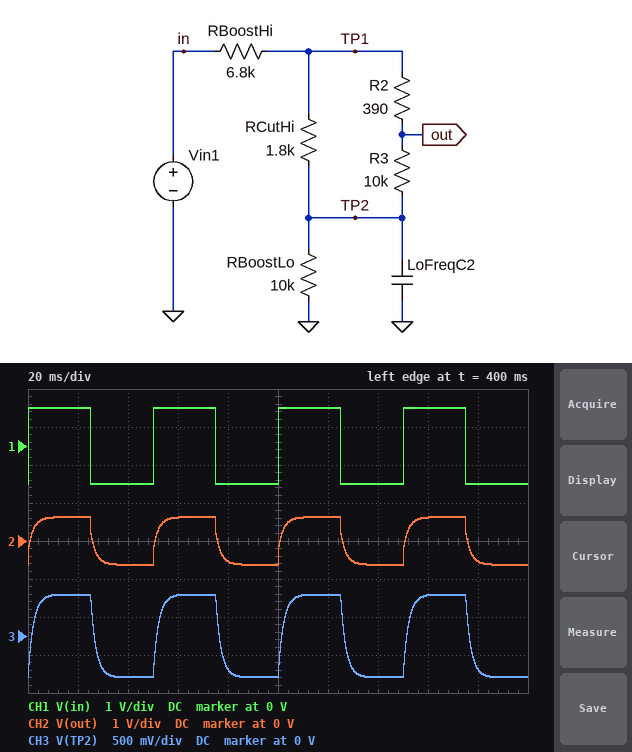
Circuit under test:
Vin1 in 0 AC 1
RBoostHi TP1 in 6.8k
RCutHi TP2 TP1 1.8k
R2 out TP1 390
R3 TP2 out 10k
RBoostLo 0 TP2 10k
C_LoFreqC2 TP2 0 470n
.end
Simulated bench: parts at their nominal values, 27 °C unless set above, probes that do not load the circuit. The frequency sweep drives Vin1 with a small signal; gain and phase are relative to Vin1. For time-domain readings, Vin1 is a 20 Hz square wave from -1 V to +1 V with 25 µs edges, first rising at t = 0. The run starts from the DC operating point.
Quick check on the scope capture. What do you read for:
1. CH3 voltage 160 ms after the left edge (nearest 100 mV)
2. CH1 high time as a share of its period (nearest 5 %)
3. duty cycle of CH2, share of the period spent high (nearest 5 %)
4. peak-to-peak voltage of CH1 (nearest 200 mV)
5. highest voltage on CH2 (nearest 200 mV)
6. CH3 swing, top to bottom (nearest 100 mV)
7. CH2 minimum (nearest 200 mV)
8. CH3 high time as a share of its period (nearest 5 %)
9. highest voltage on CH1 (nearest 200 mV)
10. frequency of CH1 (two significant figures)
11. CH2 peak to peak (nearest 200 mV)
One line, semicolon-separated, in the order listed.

500 mV; 50 %; 50 %; 2.0 V; 600 mV; 1.1 V; -600 mV; 50 %; 1.0 V; 20 Hz; 1.2 V
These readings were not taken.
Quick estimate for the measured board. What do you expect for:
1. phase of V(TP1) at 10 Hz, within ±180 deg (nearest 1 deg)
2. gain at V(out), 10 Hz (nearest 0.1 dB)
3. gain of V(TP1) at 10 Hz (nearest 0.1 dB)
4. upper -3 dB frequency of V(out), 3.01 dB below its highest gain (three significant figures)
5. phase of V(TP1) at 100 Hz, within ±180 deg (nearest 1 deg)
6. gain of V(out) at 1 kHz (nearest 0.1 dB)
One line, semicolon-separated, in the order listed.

-5 deg; -4.1 dB; -4.1 dB; 81.3 Hz; -32 deg; -14.8 dB
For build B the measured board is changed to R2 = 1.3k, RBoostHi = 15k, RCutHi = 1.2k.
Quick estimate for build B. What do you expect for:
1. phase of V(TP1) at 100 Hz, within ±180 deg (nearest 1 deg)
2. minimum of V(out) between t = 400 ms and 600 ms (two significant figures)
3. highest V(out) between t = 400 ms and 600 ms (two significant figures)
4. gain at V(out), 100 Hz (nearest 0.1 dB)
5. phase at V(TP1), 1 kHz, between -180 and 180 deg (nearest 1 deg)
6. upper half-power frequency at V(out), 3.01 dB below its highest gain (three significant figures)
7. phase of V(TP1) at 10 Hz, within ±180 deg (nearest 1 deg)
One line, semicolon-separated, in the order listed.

-45 deg; -420 mV; 420 mV; -13.6 dB; -16 deg; 56.1 Hz; -9 deg
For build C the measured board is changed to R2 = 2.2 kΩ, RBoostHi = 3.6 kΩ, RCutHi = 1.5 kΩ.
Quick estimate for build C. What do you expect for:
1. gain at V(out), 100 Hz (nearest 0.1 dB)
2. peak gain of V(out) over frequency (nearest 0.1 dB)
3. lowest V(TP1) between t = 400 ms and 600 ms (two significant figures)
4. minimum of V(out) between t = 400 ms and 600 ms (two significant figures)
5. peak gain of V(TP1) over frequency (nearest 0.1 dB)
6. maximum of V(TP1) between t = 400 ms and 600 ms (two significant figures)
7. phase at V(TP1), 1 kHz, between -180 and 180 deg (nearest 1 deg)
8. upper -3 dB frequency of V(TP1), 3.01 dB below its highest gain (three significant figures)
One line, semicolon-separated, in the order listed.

-5.1 dB; -2.6 dB; -760 mV; -740 mV; -2.4 dB; 760 mV; -10 deg; 119 Hz
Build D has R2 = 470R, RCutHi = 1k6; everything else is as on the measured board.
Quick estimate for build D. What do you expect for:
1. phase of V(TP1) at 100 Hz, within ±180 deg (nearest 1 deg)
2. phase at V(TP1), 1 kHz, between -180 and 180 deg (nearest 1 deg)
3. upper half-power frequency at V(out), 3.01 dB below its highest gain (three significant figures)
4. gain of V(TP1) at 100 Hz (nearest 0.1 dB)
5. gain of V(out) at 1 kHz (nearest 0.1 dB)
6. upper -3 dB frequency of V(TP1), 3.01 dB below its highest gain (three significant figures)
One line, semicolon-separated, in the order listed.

-33 deg; -11 deg; 80.9 Hz; -8.0 dB; -15.5 dB; 81.4 Hz
